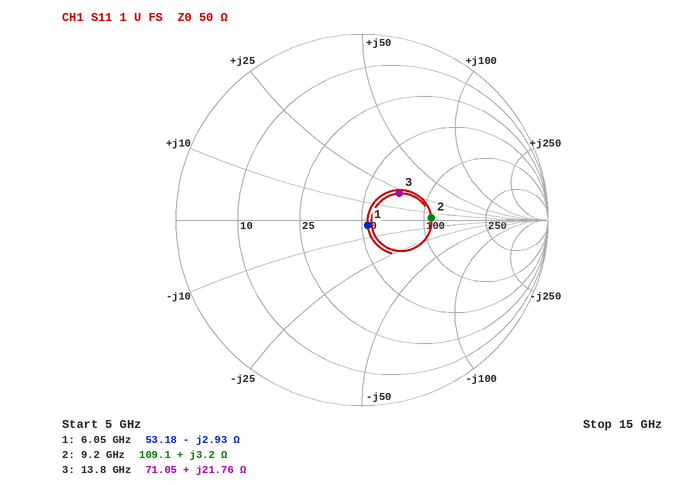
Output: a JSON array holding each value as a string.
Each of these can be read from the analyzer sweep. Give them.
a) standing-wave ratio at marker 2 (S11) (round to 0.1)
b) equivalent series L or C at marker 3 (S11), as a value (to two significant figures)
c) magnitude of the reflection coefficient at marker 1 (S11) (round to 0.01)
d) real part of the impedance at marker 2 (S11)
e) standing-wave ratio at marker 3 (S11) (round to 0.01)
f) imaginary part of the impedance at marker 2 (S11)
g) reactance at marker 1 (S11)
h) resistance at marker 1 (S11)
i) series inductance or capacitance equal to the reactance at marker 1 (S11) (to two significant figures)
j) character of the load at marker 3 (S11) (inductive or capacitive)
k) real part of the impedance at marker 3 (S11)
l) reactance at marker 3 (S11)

["2.2", "250 pH", "0.04", "109.1 Ω", "1.65", "+3.2 Ω", "-2.93 Ω", "53.18 Ω", "9.0 pF", "inductive", "71.05 Ω", "+21.76 Ω"]
